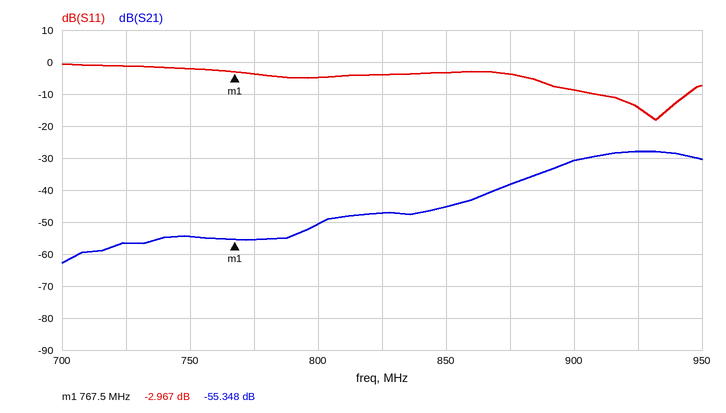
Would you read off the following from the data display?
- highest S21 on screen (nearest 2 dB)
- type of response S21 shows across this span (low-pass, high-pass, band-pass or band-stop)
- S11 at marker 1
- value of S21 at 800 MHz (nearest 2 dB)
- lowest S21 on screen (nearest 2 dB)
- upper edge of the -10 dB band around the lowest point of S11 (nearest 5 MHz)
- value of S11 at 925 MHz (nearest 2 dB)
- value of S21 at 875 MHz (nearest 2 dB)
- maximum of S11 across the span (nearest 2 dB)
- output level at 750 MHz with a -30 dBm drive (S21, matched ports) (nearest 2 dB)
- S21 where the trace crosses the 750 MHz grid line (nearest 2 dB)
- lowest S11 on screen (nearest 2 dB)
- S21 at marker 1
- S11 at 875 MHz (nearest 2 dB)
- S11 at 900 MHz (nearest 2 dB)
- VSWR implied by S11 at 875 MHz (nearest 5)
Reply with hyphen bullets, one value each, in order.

- -28 dB
- high-pass
- -2.967 dB
- -50 dB
- -62 dB
- 945 MHz
- -14 dB
- -38 dB
- 0 dB
- -84 dBm
- -54 dB
- -18 dB
- -55.348 dB
- -4 dB
- -8 dB
- 5
